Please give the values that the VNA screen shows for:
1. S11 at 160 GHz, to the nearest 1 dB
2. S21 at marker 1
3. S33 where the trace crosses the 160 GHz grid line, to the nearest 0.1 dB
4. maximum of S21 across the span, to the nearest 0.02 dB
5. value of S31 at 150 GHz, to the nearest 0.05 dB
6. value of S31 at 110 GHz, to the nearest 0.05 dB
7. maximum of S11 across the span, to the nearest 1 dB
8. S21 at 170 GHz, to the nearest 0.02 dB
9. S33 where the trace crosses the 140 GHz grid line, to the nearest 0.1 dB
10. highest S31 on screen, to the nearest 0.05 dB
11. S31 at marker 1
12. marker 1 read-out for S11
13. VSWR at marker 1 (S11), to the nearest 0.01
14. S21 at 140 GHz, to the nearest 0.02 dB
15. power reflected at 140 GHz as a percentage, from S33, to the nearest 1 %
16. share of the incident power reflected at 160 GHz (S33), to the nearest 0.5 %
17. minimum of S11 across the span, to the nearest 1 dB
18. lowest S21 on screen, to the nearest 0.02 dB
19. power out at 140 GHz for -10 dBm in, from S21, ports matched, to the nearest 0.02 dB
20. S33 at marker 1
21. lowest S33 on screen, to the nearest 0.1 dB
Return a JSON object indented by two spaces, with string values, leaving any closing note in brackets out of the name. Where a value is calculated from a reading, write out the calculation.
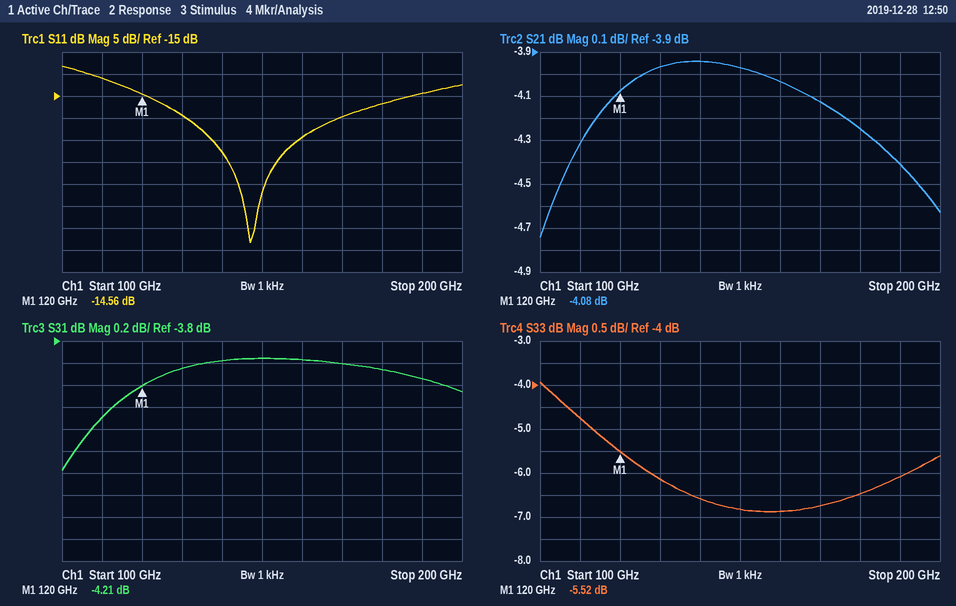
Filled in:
{
  "S11 at 160 GHz, to the nearest 1 dB": "-24 dB",
  "S21 at marker 1": "-4.08 dB",
  "S33 where the trace crosses the 160 GHz grid line, to the nearest 0.1 dB": "-6.9 dB",
  "maximum of S21 across the span, to the nearest 0.02 dB": "-3.94 dB",
  "value of S31 at 150 GHz, to the nearest 0.05 dB": "-3.95 dB",
  "value of S31 at 110 GHz, to the nearest 0.05 dB": "-4.50 dB",
  "maximum of S11 across the span, to the nearest 1 dB": "-8 dB",
  "S21 at 170 GHz, to the nearest 0.02 dB": "-4.12 dB",
  "S33 where the trace crosses the 140 GHz grid line, to the nearest 0.1 dB": "-6.6 dB",
  "highest S31 on screen, to the nearest 0.05 dB": "-3.95 dB",
  "S31 at marker 1": "-4.21 dB",
  "marker 1 read-out for S11": "-14.56 dB",
  "VSWR at marker 1 (S11), to the nearest 0.01": "(1 + 0.1871)/(1 − 0.1871) ≈ 1.46",
  "S21 at 140 GHz, to the nearest 0.02 dB": "-3.94 dB",
  "power reflected at 140 GHz as a percentage, from S33, to the nearest 1 %": "10^(-6.6/10) ≈ 22 %",
  "share of the incident power reflected at 160 GHz (S33), to the nearest 0.5 %": "10^(-6.9/10) ≈ 20.4 %, so 20.5 % to the nearest 0.5 %",
  "minimum of S11 across the span, to the nearest 1 dB": "-48 dB",
  "lowest S21 on screen, to the nearest 0.02 dB": "-4.74 dB",
  "power out at 140 GHz for -10 dBm in, from S21, ports matched, to the nearest 0.02 dB": "-10 dBm + (-3.94 dB) = -13.94 dBm",
  "S33 at marker 1": "-5.52 dB",
  "lowest S33 on screen, to the nearest 0.1 dB": "-6.9 dB"
}
